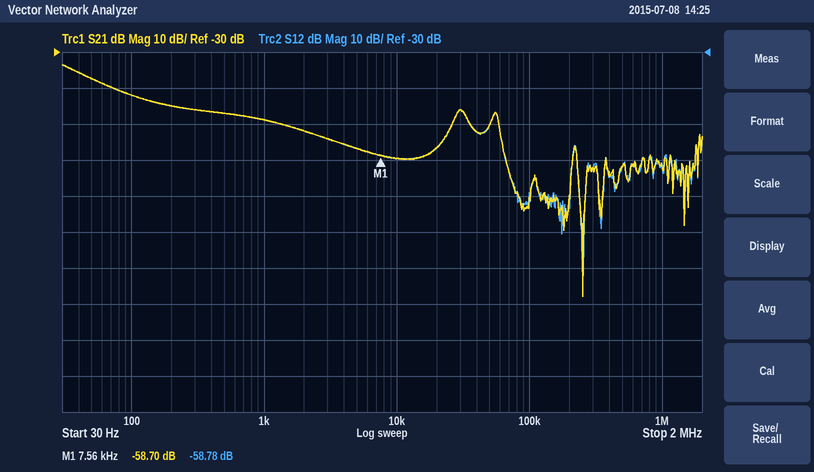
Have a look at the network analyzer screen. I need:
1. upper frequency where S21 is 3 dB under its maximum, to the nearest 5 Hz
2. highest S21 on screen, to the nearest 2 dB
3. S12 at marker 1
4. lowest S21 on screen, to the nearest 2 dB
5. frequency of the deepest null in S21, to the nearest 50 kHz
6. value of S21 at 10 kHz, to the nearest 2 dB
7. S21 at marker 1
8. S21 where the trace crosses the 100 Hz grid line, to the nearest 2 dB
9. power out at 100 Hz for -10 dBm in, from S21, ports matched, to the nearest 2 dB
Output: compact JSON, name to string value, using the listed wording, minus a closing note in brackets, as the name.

{"upper frequency where S21 is 3 dB under its maximum, to the nearest 5 Hz": "45 Hz", "highest S21 on screen, to the nearest 2 dB": "-34 dB", "S12 at marker 1": "-58.78 dB", "lowest S21 on screen, to the nearest 2 dB": "-98 dB", "frequency of the deepest null in S21, to the nearest 50 kHz": "250 kHz", "value of S21 at 10 kHz, to the nearest 2 dB": "-60 dB", "S21 at marker 1": "-58.70 dB", "S21 where the trace crosses the 100 Hz grid line, to the nearest 2 dB": "-42 dB", "power out at 100 Hz for -10 dBm in, from S21, ports matched, to the nearest 2 dB": "-52 dBm"}
